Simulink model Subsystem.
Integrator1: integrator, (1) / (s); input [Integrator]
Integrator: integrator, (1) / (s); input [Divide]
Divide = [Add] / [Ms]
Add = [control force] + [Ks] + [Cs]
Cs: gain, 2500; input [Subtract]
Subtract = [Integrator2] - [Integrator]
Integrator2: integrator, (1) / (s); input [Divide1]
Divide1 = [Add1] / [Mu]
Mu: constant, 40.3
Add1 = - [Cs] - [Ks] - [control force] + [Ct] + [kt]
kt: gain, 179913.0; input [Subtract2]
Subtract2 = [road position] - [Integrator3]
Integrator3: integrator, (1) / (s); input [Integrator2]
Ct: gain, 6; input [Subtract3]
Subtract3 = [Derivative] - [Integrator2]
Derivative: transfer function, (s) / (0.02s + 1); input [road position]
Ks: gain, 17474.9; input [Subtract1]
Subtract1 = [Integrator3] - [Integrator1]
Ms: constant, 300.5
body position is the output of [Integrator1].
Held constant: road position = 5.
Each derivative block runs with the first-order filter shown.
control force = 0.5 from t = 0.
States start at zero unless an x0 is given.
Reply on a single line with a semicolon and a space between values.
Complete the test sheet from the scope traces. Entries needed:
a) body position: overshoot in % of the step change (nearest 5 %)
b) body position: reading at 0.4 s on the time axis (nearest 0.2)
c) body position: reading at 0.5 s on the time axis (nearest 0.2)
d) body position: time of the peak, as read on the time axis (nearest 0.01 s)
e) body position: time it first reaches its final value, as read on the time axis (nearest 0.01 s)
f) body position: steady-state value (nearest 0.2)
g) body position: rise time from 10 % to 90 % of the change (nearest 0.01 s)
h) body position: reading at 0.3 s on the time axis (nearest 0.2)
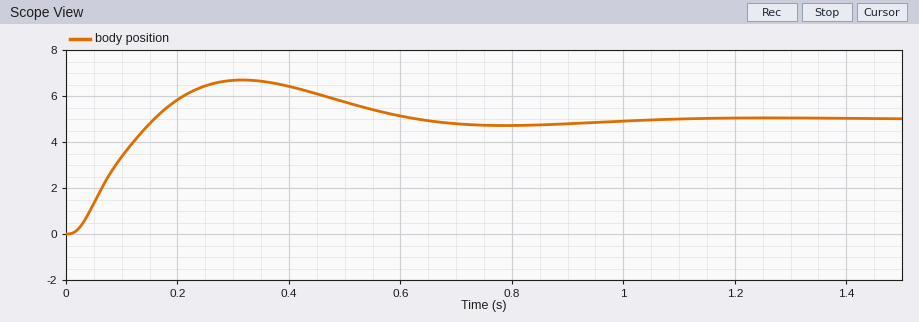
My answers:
35 %; 6.4; 5.8; 0.32 s; 0.16 s; 5.0; 0.11 s; 6.6
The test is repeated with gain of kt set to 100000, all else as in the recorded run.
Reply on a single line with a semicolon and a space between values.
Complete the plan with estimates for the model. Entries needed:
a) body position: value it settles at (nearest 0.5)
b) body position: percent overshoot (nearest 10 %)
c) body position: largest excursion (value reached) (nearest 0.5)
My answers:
5.0; 40 %; 7.0
